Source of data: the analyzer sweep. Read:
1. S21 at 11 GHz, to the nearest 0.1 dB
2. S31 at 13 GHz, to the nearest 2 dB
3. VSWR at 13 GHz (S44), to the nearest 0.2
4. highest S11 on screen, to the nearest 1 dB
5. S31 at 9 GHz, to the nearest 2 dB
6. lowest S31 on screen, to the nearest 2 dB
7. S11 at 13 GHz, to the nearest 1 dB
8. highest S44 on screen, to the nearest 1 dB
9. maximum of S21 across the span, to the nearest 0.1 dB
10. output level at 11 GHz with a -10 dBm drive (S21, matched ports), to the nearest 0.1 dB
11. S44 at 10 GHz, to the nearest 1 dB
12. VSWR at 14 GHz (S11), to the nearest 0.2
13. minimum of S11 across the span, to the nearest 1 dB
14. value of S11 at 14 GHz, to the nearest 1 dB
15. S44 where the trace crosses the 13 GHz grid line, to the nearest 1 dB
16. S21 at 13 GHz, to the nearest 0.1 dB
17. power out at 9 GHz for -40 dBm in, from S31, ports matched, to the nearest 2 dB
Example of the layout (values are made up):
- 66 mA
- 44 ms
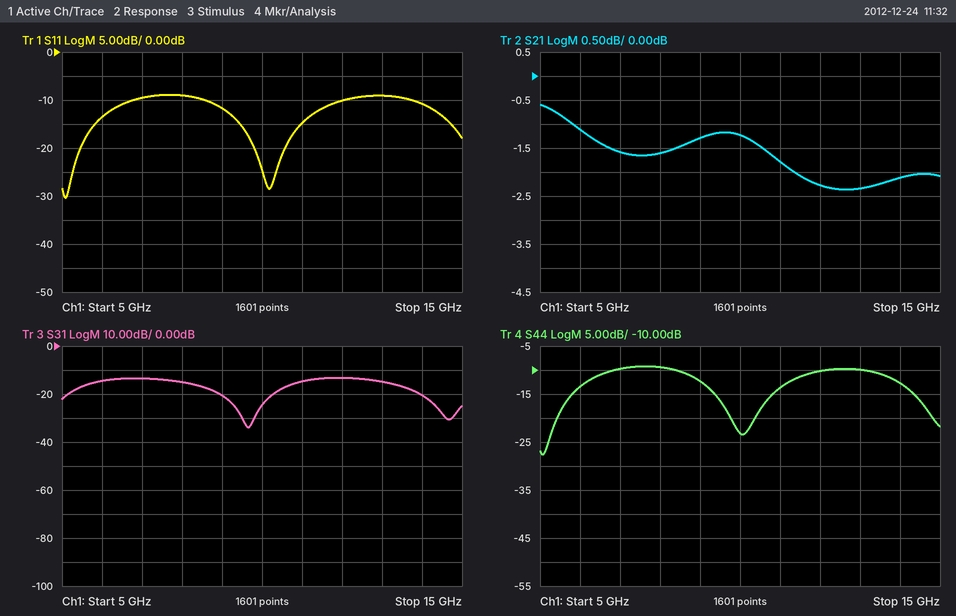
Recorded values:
- -1.8 dB
- -14 dB
- 2.0
- -9 dB
- -20 dB
- -34 dB
- -9 dB
- -9 dB
- -0.6 dB
- -11.8 dBm
- -23 dB
- 1.8
- -30 dB
- -11 dB
- -10 dB
- -2.3 dB
- -60 dBm
